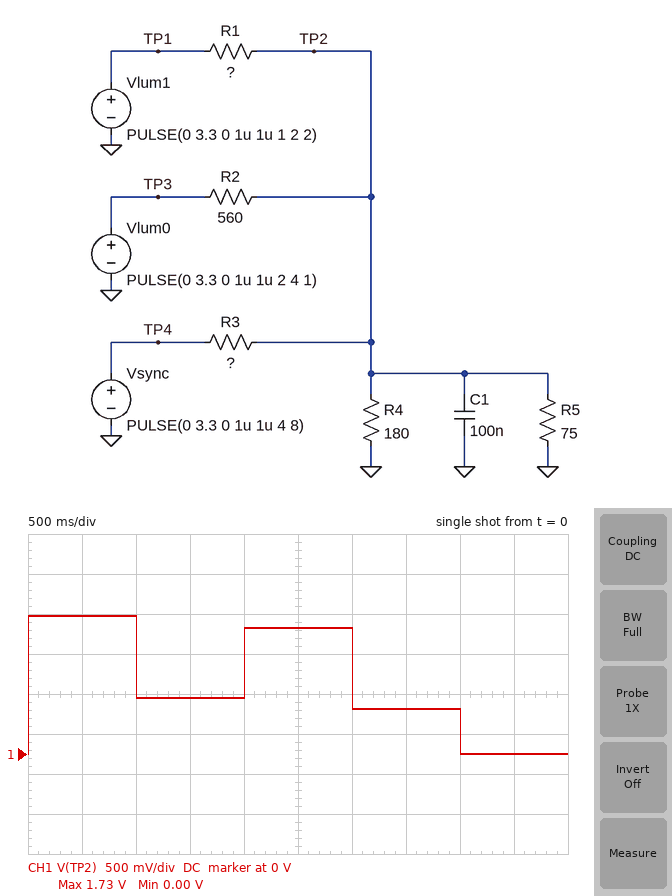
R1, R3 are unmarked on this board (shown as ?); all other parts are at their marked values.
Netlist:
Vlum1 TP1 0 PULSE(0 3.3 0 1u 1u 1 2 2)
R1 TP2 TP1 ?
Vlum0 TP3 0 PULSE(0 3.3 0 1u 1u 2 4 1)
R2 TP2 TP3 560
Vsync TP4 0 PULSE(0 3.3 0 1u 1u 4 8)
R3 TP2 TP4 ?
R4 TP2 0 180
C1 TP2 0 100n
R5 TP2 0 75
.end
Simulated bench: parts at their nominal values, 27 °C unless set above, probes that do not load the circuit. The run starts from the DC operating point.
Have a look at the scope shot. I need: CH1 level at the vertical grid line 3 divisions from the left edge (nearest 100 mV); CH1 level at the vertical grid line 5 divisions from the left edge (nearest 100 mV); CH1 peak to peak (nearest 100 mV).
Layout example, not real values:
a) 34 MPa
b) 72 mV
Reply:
a) 700 mV
b) 1.6 V
c) 1.7 V
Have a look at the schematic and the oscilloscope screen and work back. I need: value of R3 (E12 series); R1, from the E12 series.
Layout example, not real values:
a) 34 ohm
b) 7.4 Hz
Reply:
a) 150 Ω
b) 82 Ω
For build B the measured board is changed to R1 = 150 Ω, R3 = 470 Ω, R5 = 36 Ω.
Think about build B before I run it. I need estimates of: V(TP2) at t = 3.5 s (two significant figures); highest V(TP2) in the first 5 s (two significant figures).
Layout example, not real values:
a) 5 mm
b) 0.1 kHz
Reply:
a) 160 mV
b) 800 mV
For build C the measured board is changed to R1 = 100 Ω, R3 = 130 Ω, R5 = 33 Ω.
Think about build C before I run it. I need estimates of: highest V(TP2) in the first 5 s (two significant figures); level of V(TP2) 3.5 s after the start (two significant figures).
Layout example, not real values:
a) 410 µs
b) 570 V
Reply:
a) 1.2 V
b) 460 mV
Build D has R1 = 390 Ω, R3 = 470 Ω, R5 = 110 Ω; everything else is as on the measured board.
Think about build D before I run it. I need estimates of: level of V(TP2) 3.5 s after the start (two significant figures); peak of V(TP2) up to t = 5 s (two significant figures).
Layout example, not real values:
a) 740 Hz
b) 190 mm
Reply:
a) 330 mV
b) 1.0 V
